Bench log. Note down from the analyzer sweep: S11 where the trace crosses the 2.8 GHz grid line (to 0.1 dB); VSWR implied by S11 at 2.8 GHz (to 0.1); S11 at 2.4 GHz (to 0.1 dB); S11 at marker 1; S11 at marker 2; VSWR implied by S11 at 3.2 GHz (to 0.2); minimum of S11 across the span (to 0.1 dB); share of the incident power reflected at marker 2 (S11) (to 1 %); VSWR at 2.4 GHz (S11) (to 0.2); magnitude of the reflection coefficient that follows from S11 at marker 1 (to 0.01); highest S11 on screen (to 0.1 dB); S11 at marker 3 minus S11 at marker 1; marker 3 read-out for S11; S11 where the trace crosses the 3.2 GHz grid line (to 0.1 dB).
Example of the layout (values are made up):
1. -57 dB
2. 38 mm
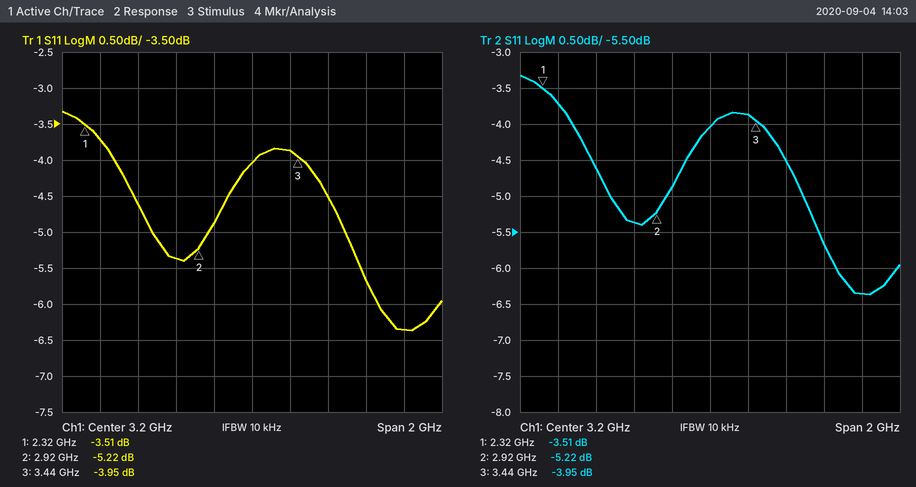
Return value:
1. -5.4 dB
2. 3.3
3. -3.7 dB
4. -3.51 dB
5. -5.22 dB
6. 4.4
7. -6.4 dB
8. 30 %
9. 4.8
10. 0.67
11. -3.3 dB
12. -0.44 dB
13. -3.95 dB
14. -4.0 dB
